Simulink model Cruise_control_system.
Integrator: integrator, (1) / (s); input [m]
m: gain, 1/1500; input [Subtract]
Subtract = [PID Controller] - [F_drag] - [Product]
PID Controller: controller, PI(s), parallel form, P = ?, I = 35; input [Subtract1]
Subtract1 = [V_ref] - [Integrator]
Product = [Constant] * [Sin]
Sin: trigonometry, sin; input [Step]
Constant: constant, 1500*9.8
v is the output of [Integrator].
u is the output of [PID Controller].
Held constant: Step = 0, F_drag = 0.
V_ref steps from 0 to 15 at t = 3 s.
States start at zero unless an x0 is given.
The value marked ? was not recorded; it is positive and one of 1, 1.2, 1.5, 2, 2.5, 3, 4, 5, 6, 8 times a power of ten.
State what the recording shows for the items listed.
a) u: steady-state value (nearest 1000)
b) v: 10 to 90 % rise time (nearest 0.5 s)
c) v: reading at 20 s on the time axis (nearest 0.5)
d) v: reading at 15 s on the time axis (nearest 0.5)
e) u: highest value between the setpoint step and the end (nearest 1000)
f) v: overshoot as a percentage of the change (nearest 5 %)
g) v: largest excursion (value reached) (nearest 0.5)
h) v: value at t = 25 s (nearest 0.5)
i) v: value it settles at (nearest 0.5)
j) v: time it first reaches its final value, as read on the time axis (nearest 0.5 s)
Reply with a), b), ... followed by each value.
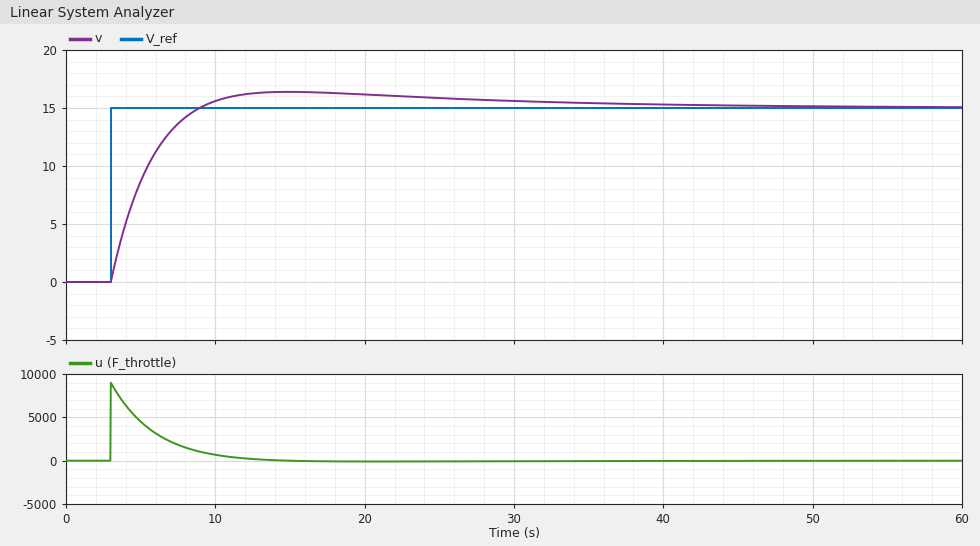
a) 0
b) 4.0 s
c) 16.0
d) 16.5
e) 9000
f) 10 %
g) 16.5
h) 16.0
i) 15.0
j) 9.0 s
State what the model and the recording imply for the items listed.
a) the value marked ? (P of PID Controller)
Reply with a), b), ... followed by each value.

a) 600
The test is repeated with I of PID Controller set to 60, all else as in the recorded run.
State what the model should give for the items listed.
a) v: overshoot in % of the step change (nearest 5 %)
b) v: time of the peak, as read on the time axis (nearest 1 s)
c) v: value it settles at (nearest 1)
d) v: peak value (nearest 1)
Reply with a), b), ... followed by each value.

a) 15 %
b) 13 s
c) 15
d) 17
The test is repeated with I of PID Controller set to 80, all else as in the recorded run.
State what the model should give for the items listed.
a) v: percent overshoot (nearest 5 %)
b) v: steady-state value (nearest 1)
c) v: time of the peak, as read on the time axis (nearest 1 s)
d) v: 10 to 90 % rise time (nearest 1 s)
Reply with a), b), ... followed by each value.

a) 15 %
b) 15
c) 12 s
d) 3 s
